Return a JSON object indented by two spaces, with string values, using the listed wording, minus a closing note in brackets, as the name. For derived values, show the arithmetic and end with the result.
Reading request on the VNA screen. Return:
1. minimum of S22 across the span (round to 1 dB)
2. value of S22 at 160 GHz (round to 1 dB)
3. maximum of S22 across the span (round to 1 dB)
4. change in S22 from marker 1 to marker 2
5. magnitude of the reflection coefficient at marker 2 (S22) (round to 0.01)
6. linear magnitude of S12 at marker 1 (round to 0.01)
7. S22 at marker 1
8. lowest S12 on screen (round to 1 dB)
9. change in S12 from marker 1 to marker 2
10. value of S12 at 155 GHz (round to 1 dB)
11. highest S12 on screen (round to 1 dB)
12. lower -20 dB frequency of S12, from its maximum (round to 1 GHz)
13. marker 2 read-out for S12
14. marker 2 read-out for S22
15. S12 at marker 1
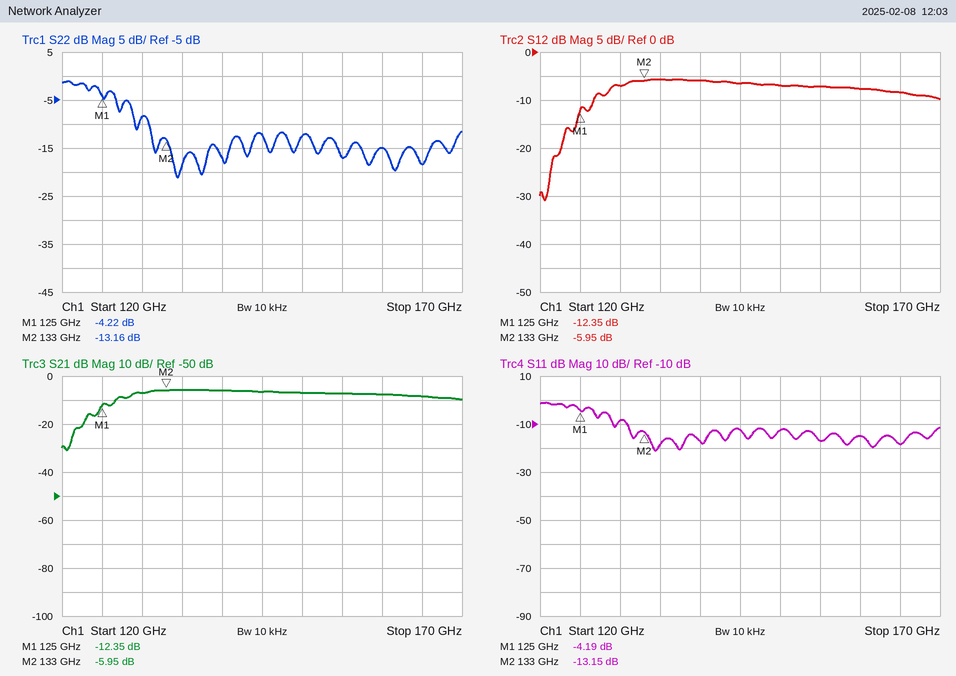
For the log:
{
  "minimum of S22 across the span": "-21 dB",
  "value of S22 at 160 GHz": "-15 dB",
  "maximum of S22 across the span": "-1 dB",
  "change in S22 from marker 1 to marker 2": "-13.16 − (-4.22) = -8.94 dB",
  "magnitude of the reflection coefficient at marker 2 (S22)": "10^(-13.16/20) ≈ 0.22",
  "linear magnitude of S12 at marker 1": "10^(-12.35/20) ≈ 0.24",
  "S22 at marker 1": "-4.22 dB",
  "lowest S12 on screen": "-31 dB",
  "change in S12 from marker 1 to marker 2": "-5.95 − (-12.35) = 6.40 dB",
  "value of S12 at 155 GHz": "-7 dB",
  "highest S12 on screen": "-6 dB",
  "lower -20 dB frequency of S12, from its maximum": "121 GHz",
  "marker 2 read-out for S12": "-5.95 dB",
  "marker 2 read-out for S22": "-13.16 dB",
  "S12 at marker 1": "-12.35 dB"
}
